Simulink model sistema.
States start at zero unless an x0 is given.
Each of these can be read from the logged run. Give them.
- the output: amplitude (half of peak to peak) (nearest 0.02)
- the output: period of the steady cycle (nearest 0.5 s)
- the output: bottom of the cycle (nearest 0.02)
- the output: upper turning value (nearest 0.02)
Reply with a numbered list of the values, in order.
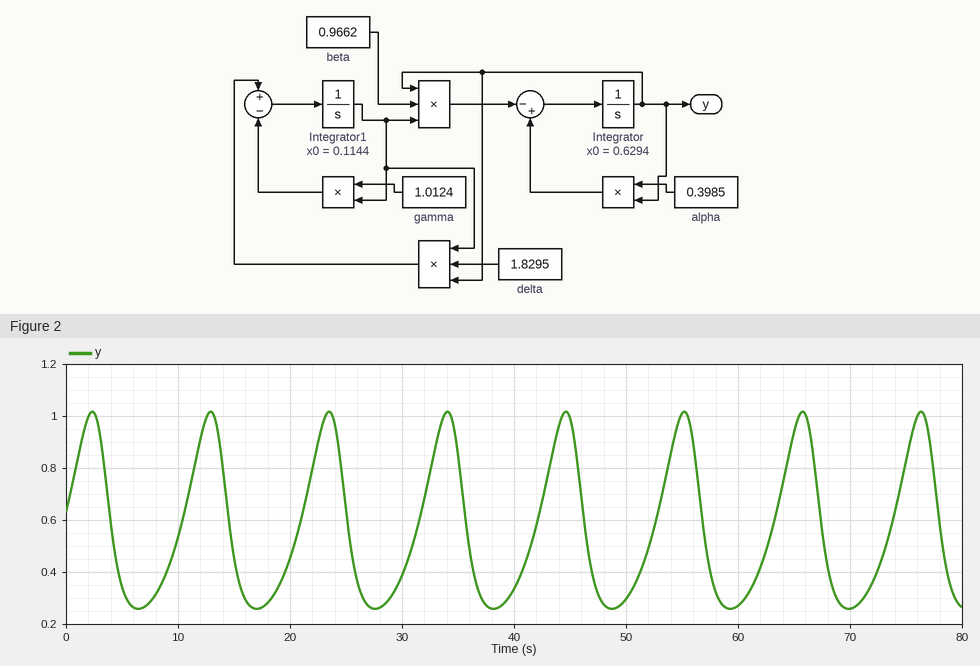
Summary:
1. 0.38
2. 10.5 s
3. 0.26
4. 1.02
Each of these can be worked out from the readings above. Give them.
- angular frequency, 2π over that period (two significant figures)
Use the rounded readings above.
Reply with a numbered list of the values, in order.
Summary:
1. 0.60 rad/s
